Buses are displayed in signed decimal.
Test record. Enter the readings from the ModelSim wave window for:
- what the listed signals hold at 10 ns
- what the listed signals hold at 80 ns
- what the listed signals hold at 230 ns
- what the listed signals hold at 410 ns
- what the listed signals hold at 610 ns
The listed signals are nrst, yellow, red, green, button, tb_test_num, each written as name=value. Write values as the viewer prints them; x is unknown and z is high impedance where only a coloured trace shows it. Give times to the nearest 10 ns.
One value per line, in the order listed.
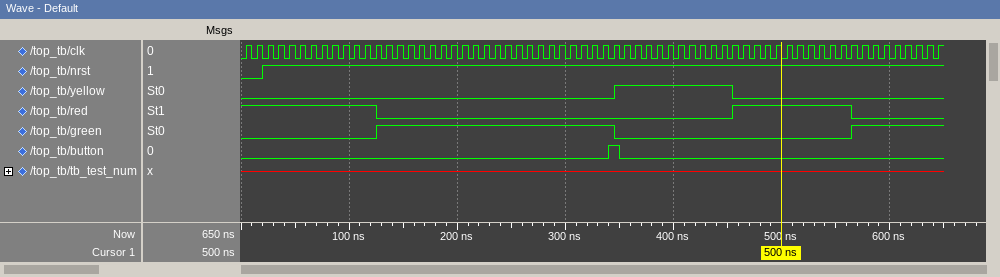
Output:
nrst=0, yellow=0, red=1, green=0, button=0, tb_test_num=x
nrst=1, yellow=0, red=1, green=0, button=0, tb_test_num=x
nrst=1, yellow=0, red=0, green=1, button=0, tb_test_num=x
nrst=1, yellow=1, red=0, green=0, button=0, tb_test_num=x
nrst=1, yellow=0, red=0, green=1, button=0, tb_test_num=x
